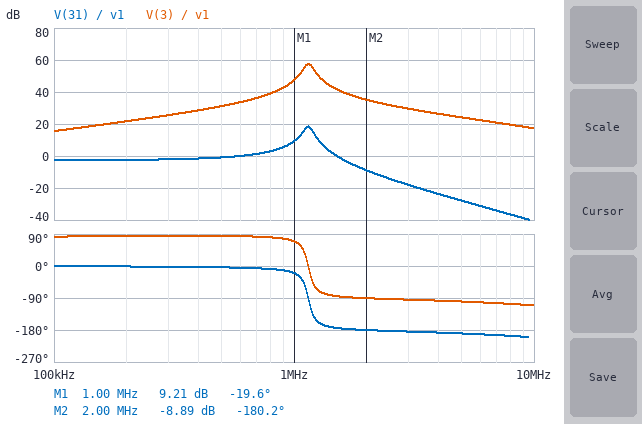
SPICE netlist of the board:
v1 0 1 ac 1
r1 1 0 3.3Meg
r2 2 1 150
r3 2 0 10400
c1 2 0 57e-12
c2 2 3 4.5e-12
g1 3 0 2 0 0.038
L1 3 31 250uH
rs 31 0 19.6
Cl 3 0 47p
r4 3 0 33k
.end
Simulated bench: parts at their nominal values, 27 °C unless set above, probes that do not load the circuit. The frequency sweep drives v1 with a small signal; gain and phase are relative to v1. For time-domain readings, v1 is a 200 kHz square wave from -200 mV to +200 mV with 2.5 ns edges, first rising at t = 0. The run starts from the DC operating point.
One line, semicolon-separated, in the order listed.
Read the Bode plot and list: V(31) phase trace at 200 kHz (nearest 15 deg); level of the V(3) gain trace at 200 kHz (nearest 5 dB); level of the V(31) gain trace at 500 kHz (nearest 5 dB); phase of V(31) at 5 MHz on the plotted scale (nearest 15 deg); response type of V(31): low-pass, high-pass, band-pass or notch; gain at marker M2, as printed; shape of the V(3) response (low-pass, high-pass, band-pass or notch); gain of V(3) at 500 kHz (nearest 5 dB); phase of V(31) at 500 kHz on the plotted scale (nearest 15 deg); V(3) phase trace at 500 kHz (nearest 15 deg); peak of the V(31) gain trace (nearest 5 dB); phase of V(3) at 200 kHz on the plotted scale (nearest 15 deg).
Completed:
0 deg; 20 dB; 0 dB; -195 deg; low-pass; -8.89 dB; band-pass; 30 dB; 0 deg; 90 deg; 20 dB; 90 deg
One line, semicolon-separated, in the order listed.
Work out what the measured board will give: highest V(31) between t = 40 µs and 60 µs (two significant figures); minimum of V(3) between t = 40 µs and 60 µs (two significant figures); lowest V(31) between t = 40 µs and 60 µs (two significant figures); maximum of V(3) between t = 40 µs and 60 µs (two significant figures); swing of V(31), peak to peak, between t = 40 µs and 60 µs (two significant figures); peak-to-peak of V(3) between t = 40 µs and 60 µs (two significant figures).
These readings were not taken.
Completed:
340 mV; -19 V; -340 mV; 19 V; 680 mV; 38 V
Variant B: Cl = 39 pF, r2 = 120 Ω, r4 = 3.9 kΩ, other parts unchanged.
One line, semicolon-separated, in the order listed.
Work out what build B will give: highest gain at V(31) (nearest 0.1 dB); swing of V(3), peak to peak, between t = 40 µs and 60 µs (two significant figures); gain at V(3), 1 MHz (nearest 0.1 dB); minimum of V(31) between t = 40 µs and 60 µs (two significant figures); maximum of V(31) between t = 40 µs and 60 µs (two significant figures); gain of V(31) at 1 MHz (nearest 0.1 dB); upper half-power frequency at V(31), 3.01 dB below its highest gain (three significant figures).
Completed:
3.1 dB; 41 V; 40.4 dB; -270 mV; 270 mV; 2.3 dB; 1.47 MHz
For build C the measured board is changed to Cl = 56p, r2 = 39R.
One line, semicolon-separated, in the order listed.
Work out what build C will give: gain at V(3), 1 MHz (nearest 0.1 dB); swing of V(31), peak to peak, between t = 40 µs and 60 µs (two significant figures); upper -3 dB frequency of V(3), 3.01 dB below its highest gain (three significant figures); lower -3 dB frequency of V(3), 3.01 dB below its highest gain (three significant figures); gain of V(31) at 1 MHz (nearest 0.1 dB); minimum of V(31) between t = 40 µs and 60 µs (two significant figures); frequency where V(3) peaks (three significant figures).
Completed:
44.8 dB; 650 mV; 1.27 MHz; 1.19 MHz; 6.7 dB; -330 mV; 1.23 MHz
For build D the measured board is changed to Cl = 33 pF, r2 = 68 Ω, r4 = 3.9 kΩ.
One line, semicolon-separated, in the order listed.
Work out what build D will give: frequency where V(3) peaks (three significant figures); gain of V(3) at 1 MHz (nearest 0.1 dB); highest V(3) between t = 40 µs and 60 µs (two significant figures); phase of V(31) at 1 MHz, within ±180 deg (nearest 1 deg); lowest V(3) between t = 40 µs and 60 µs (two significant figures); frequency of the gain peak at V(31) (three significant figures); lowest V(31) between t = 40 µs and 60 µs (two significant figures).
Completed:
1.44 MHz; 39.0 dB; 23 V; -40 deg; -23 V; 1.30 MHz; -260 mV
